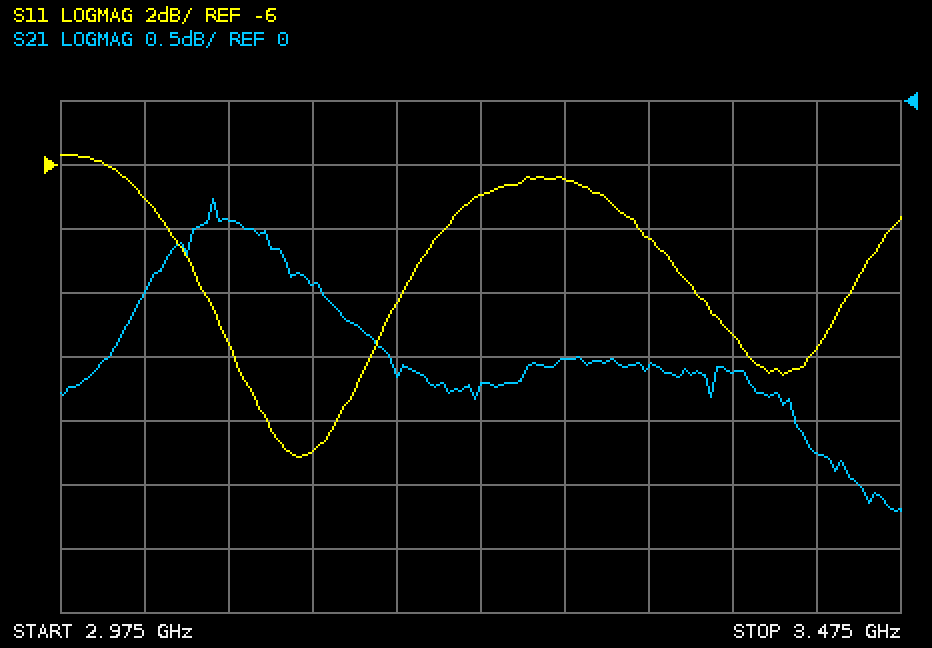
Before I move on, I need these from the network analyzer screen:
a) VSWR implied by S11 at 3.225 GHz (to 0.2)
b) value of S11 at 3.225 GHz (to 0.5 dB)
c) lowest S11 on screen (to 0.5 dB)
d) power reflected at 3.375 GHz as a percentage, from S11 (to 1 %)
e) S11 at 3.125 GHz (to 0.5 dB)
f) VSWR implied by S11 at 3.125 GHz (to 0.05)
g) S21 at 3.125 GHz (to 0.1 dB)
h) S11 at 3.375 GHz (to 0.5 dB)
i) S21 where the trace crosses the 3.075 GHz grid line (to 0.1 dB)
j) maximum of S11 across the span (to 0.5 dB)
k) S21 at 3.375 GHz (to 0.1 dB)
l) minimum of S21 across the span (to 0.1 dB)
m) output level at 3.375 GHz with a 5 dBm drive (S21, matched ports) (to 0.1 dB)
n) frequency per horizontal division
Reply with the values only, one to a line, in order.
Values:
2.6
-7.0 dB
-15.0 dB
7 %
-15.0 dB
1.45
-1.4 dB
-11.5 dB
-0.9 dB
-5.5 dB
-2.1 dB
-3.2 dB
2.9 dBm
50 MHz
